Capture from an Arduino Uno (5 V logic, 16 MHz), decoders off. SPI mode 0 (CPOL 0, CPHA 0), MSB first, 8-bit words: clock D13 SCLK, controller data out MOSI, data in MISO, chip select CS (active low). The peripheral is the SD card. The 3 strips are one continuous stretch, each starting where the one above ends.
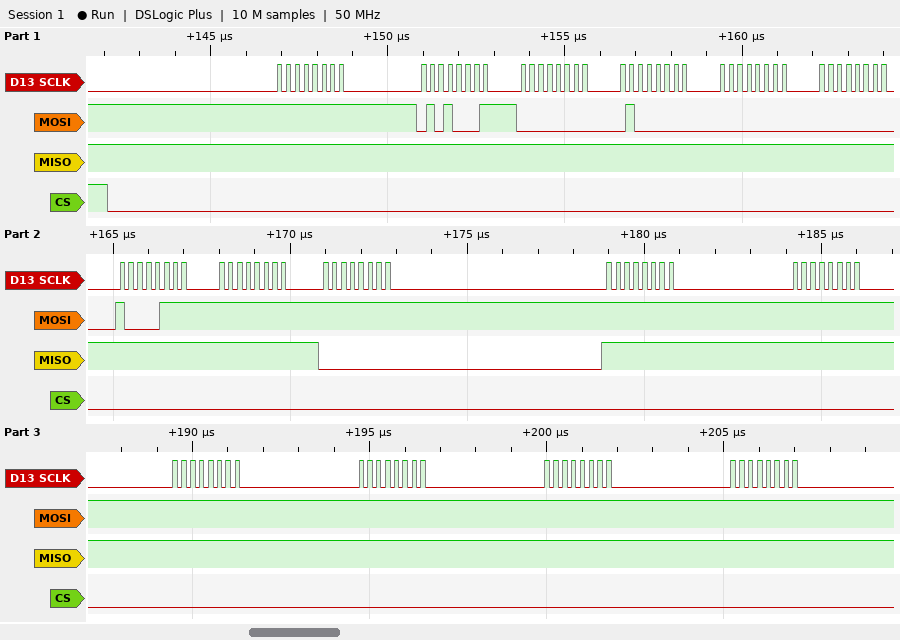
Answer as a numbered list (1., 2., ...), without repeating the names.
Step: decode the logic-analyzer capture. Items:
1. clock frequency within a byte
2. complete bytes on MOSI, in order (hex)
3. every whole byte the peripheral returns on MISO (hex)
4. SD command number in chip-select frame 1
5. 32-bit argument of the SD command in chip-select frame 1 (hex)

1. 4 MHz
2. FF 51 00 40 00 00 87 FF FF FF FF FF FF FF FF
3. FF FF FF FF FF FF FF FF 00 FF FF FF FF FF FF
4. CMD17
5. 0x00400000
